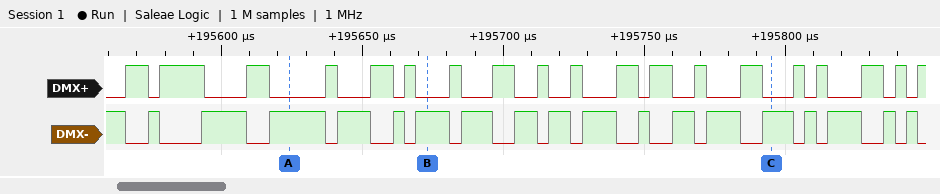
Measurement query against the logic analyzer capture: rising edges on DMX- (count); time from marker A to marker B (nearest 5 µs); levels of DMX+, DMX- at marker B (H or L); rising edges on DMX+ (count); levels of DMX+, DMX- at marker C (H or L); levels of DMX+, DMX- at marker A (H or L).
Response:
18
50 µs
DMX+=L, DMX-=H
19
DMX+=L, DMX-=H
DMX+=L, DMX-=H
